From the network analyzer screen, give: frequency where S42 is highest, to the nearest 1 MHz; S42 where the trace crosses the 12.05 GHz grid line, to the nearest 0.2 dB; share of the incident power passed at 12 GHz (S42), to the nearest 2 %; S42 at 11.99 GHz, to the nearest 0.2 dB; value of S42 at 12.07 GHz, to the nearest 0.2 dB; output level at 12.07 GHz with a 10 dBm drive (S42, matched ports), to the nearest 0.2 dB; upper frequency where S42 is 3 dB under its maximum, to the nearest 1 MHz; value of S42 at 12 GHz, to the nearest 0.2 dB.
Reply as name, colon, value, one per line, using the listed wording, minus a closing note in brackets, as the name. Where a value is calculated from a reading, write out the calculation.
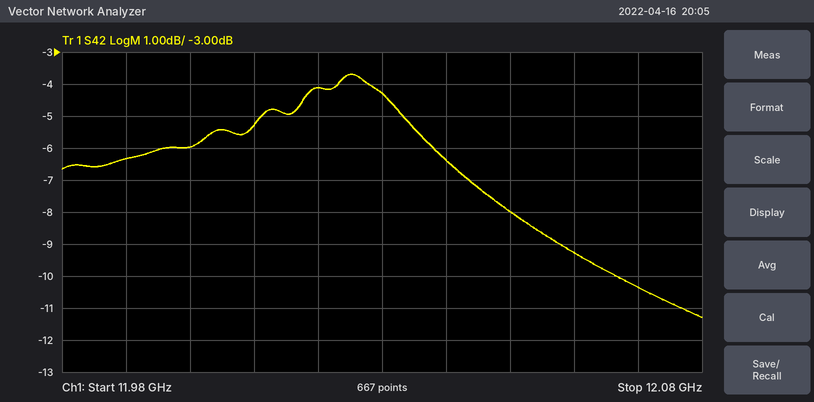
frequency where S42 is highest, to the nearest 1 MHz: 12.025 GHz
S42 where the trace crosses the 12.05 GHz grid line, to the nearest 0.2 dB: -8.0 dB
share of the incident power passed at 12 GHz (S42), to the nearest 2 %: 10^(-6/10) ≈ 25.1 %, so 26 % to the nearest 2 %
S42 at 11.99 GHz, to the nearest 0.2 dB: -6.4 dB
value of S42 at 12.07 GHz, to the nearest 0.2 dB: -10.4 dB
output level at 12.07 GHz with a 10 dBm drive (S42, matched ports), to the nearest 0.2 dB: 10 dBm + (-10.4 dB) = -0.4 dBm
upper frequency where S42 is 3 dB under its maximum, to the nearest 1 MHz: 12.042 GHz
value of S42 at 12 GHz, to the nearest 0.2 dB: -6.0 dB
